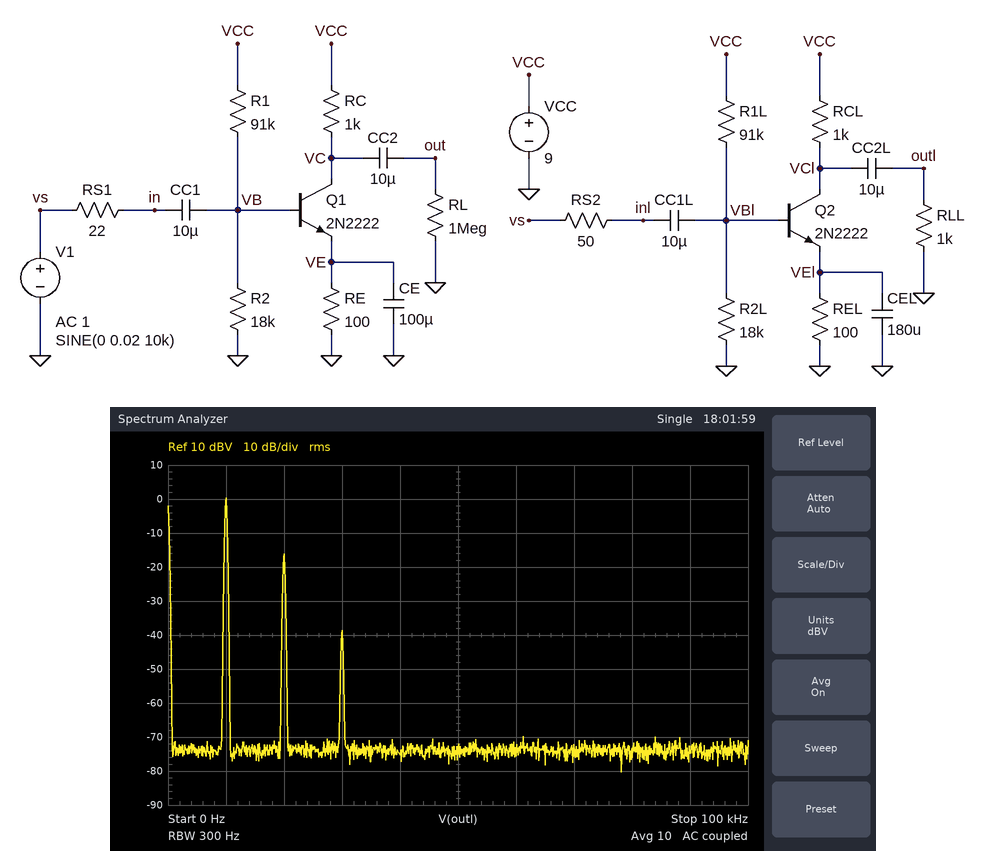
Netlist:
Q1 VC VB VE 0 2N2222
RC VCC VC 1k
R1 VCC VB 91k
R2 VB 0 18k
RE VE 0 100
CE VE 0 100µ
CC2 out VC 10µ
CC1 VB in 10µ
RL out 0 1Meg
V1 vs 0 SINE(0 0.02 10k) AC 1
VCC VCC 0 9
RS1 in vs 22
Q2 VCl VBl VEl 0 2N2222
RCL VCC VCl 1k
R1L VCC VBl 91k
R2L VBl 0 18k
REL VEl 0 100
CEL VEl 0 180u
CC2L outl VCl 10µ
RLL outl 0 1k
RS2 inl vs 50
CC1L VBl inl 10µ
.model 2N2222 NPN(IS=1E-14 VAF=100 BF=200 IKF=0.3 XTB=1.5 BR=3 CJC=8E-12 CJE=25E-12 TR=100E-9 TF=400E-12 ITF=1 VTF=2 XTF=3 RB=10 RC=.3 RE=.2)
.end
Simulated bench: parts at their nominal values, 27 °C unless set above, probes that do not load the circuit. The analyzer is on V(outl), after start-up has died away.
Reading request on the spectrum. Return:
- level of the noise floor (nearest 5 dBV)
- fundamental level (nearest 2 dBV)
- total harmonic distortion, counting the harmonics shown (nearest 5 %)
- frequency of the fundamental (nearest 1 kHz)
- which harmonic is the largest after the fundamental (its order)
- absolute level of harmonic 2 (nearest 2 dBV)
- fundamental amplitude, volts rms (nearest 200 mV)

-75 dBV
0 dBV
15 %
10 kHz
2
-16 dBV
1.0 V
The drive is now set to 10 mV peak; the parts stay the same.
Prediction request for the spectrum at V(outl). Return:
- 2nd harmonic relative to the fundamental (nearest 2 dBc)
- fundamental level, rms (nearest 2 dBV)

-22 dBc
-6 dBV
